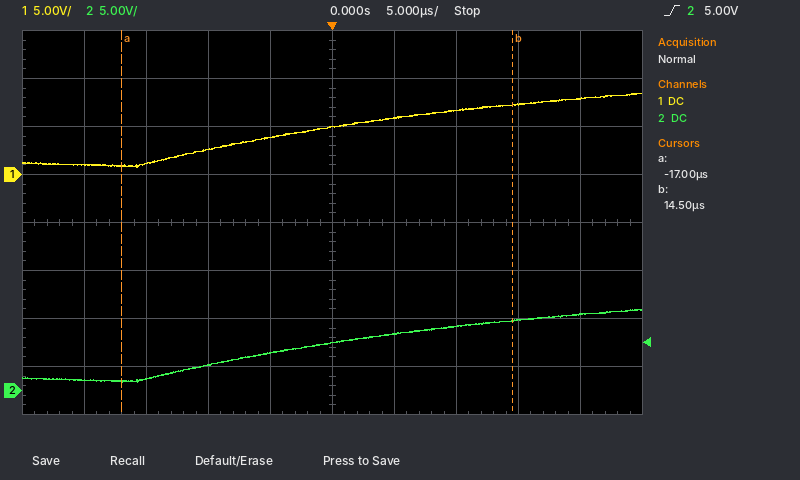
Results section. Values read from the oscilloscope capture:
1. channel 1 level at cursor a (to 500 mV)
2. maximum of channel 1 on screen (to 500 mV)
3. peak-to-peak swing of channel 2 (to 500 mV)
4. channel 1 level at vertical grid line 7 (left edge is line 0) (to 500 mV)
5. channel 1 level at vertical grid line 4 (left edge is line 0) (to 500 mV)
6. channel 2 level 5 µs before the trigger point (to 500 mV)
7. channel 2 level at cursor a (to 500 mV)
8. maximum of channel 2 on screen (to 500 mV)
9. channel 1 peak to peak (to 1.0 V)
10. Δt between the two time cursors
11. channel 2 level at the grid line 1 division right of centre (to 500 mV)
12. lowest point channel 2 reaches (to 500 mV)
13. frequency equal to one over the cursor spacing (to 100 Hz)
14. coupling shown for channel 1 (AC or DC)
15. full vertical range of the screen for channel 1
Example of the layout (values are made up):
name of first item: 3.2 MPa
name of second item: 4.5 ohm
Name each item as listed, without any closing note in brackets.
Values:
channel 1 level at cursor a: 1.0 V
maximum of channel 1 on screen: 8.5 V
peak-to-peak swing of channel 2: 7.5 V
channel 1 level at vertical grid line 7 (left edge is line 0): 6.5 V
channel 1 level at vertical grid line 4 (left edge is line 0): 4.0 V
channel 2 level 5 µs before the trigger point: 4.0 V
channel 2 level at cursor a: 1.0 V
maximum of channel 2 on screen: 8.5 V
channel 1 peak to peak: 8.0 V
Δt between the two time cursors: 31.5 µs
channel 2 level at the grid line 1 division right of centre: 6.0 V
lowest point channel 2 reaches: 1.0 V
frequency equal to one over the cursor spacing: 31.7 kHz
coupling shown for channel 1: DC
full vertical range of the screen for channel 1: 40 V
